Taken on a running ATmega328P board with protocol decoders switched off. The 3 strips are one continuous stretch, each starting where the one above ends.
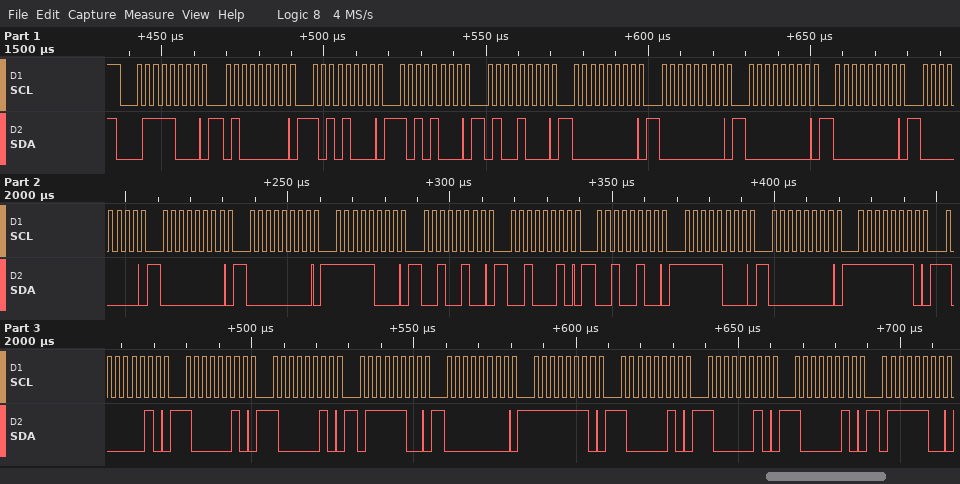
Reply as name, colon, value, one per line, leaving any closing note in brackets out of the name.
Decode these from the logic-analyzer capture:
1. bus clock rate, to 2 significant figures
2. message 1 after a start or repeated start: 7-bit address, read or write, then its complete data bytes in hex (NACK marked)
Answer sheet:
bus clock rate, to 2 significant figures: 400 kHz
message 1 after a start or repeated start: 7-bit address, read or write, then its complete data bytes in hex: 0x3C write: 40 A8 A8 48 00 00 00 00 00 00 00 F8 24 22 24 F8 00 FE 82 82 82 7C 00 FE 82 82 82 7C
